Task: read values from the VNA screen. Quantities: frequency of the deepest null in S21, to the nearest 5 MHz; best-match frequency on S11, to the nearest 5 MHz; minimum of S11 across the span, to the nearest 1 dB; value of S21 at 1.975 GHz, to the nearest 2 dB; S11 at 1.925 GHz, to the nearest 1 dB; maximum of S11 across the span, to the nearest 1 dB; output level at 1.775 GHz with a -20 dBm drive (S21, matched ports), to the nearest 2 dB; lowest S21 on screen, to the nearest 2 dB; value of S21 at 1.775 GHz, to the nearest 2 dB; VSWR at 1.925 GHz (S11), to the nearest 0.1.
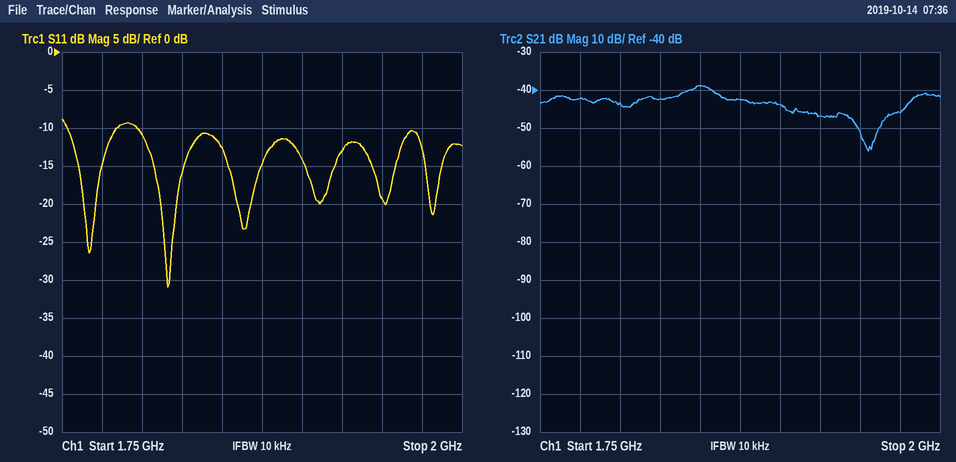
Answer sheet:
1.955 GHz
1.815 GHz
-31 dB
-46 dB
-13 dB
-9 dB
-62 dBm
-56 dB
-42 dB
1.6
